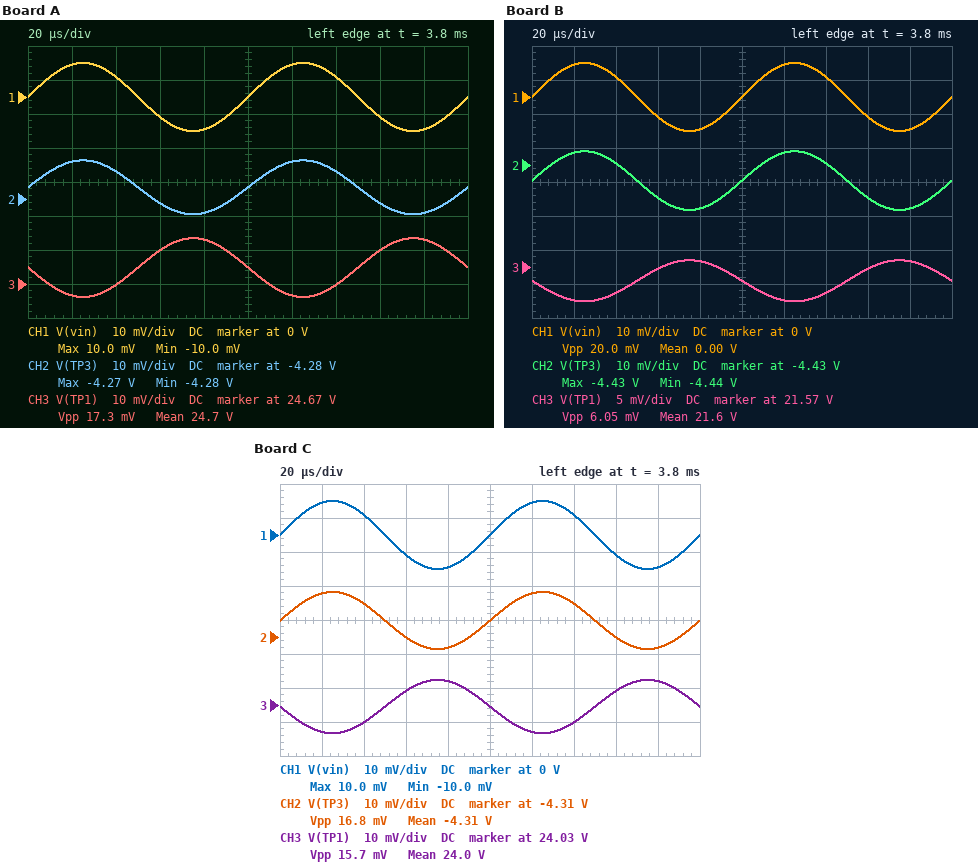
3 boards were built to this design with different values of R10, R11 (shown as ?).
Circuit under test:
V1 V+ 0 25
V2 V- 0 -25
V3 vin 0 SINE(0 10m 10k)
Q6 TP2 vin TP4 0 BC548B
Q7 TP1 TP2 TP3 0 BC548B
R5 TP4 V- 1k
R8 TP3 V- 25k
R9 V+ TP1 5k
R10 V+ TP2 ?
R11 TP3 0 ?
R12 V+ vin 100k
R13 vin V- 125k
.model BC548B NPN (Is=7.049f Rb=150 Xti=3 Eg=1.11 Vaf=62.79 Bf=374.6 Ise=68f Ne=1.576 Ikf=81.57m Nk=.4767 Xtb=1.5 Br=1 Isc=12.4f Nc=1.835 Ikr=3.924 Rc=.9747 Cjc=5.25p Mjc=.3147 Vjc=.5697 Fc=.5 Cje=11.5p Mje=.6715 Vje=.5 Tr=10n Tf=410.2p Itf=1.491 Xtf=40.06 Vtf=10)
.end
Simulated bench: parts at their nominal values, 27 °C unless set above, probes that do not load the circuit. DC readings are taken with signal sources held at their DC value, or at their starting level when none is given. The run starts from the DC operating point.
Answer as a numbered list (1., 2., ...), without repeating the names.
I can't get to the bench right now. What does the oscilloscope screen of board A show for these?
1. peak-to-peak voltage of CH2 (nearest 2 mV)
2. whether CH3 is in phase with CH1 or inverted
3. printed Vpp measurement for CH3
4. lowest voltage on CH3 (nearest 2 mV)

1. 16 mV
2. inverted
3. 17.3 mV
4. 24.666 V
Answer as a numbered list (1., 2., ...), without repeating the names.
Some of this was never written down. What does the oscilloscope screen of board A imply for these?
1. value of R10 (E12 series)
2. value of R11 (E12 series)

1. 18 kΩ
2. 5.6 kΩ
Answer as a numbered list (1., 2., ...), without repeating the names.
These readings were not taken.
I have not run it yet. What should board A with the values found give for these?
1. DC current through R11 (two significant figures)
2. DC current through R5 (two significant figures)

1. 760 µA
2. 21 mA
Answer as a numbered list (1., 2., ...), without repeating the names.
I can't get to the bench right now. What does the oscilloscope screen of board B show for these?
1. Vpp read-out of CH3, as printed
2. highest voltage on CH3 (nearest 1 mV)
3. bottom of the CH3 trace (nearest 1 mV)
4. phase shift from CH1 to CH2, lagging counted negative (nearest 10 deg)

1. 6.05 mV
2. 21.571 V
3. 21.565 V
4. 0 deg
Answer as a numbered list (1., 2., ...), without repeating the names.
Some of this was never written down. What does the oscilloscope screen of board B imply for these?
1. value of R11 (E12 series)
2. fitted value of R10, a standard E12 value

1. 33 kΩ
2. 33 kΩ
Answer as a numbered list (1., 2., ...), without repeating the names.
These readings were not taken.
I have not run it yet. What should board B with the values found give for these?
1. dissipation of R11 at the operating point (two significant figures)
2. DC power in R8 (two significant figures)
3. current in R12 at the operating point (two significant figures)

1. 600 µW
2. 17 mW
3. 250 µA
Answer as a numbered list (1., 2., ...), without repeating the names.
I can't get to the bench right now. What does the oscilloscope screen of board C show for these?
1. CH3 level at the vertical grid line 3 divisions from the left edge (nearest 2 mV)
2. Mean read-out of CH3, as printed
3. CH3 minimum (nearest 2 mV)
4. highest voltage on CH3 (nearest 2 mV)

1. 24.034 V
2. 24.0 V
3. 24.022 V
4. 24.038 V
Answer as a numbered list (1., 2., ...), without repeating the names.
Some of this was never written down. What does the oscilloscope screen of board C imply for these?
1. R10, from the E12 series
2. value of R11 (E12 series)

1. 18 kΩ
2. 6.8 kΩ
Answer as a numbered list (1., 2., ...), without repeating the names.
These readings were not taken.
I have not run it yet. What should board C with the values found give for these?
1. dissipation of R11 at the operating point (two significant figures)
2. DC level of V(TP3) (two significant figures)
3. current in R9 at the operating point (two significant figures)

1. 2.7 mW
2. -4.3 V
3. 190 µA
